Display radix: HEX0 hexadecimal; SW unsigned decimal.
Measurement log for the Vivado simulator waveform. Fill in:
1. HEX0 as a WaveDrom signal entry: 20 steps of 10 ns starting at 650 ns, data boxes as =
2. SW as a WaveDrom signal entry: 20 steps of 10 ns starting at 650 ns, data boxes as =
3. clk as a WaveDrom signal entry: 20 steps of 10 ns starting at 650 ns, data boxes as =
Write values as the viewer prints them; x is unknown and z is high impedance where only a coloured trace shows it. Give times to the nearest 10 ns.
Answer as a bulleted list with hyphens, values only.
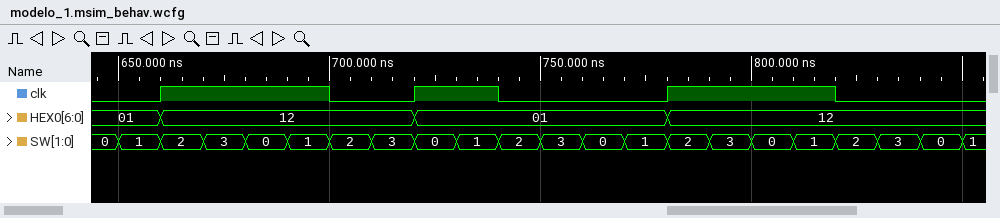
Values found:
- {name: 'HEX0', wave: '==.....=.....=......', data: '01 12 01 12'}
- {name: 'SW', wave: '====================', data: '1 2 3 0 1 2 3 0 1 2 3 0 1 2 3 0 1 2 3 0'}
- {name: 'clk', wave: '01...0.1.0...1...0..'}
